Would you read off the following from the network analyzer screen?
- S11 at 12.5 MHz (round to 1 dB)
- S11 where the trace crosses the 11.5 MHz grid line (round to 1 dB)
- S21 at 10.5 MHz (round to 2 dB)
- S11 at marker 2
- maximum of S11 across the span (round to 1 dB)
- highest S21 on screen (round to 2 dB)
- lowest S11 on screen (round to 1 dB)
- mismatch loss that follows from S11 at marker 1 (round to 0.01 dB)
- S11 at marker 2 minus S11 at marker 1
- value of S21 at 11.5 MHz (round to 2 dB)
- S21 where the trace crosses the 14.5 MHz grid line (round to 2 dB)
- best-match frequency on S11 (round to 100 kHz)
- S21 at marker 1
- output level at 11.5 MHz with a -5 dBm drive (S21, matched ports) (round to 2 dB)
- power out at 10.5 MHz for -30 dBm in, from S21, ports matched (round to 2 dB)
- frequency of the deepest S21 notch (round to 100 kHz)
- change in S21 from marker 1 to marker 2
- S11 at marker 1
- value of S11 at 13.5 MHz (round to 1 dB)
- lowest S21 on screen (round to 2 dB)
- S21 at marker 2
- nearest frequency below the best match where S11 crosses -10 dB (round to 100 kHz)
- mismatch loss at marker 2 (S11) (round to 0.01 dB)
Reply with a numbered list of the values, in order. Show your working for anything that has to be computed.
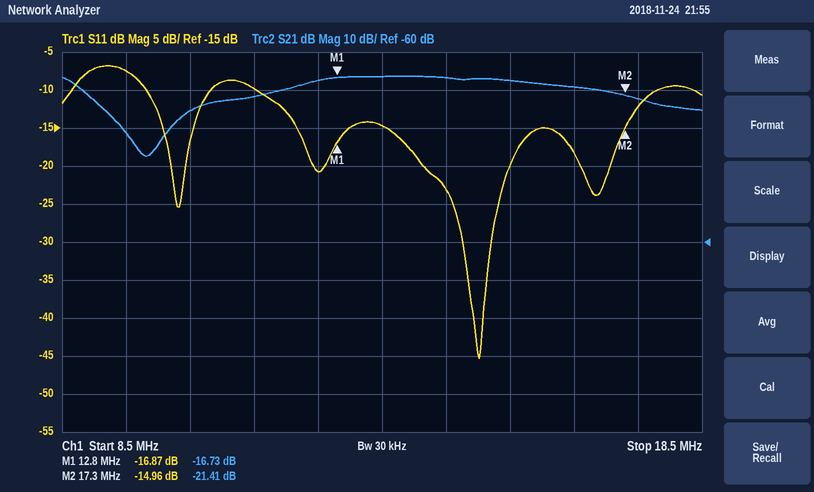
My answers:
1. -21 dB
2. -10 dB
3. -26 dB
4. -14.96 dB
5. -7 dB
6. -16 dB
7. -45 dB
8. −10 log10(1 − 10^(-16.87/10)) ≈ 0.09 dB
9. -14.96 − (-16.87) = 1.91 dB
10. -22 dB
11. -16 dB
12. 15.0 MHz
13. -16.73 dB
14. -5 dBm + (-22 dB) = -26 dBm
15. -30 dBm + (-26 dB) = -56 dBm
16. 9.8 MHz
17. -21.41 − (-16.73) = -4.68 dB
18. -16.87 dB
19. -15 dB
20. -38 dB
21. -21.41 dB
22. 11.5 MHz
23. −10 log10(1 − 10^(-14.96/10)) ≈ 0.14 dB
